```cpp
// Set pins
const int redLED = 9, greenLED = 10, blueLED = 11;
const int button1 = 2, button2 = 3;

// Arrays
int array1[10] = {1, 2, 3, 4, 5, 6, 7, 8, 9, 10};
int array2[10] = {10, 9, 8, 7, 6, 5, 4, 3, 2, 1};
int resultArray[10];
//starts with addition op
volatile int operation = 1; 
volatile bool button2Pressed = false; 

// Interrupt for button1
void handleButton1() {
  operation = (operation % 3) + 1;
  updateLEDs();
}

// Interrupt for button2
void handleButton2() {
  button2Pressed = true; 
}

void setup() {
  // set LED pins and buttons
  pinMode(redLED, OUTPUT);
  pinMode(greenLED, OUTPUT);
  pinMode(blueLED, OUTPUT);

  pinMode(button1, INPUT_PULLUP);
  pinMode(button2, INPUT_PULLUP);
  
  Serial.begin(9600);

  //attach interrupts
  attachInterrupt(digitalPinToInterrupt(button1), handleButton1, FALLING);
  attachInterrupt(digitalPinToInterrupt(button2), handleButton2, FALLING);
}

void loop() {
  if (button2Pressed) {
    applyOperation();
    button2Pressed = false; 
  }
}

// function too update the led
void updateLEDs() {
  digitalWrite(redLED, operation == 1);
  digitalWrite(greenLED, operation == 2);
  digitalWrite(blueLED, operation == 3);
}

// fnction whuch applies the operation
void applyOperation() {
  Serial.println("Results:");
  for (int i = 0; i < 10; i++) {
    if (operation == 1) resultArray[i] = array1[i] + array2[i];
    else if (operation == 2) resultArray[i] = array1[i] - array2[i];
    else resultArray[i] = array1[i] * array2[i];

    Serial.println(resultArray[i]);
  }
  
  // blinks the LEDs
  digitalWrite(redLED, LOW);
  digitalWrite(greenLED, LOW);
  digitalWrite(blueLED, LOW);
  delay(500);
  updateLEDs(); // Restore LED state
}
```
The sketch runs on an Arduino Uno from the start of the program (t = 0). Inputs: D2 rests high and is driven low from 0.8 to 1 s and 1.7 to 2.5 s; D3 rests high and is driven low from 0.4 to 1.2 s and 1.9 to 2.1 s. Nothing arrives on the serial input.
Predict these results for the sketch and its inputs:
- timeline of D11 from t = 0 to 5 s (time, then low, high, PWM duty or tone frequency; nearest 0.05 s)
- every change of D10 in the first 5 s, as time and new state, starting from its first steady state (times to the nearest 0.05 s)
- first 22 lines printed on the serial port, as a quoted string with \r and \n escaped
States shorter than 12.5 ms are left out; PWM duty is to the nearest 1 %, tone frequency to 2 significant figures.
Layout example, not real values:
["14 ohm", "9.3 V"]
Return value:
["0 s low; 1.7 s high; 1.9 s low; 2.4 s high", "0 s low; 0.8 s high; 1.7 s low", "\"Results:\\r\\n11\\r\\n11\\r\\n11\\r\\n11\\r\\n11\\r\\n11\\r\\n11\\r\\n11\\r\\n11\\r\\n11\\r\\nResults:\\r\\n10\\r\\n18\\r\\n24\\r\\n28\\r\\n30\\r\\n30\\r\\n28\\r\\n24\\r\\n18\\r\\n10\\r\\n\""]
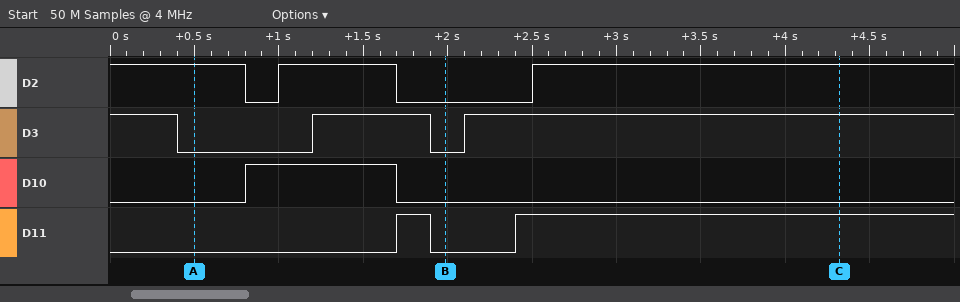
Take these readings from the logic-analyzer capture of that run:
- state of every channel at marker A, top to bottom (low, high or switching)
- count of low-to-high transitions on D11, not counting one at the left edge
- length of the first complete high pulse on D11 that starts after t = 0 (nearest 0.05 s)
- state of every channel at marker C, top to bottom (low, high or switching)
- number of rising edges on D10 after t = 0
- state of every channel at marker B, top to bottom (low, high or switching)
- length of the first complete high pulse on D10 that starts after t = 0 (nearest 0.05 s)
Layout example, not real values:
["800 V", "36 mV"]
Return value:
["D2 high, D3 low, D10 low, D11 low", "2", "0.20 s", "D2 high, D3 high, D10 low, D11 high", "1", "D2 low, D3 low, D10 low, D11 low", "0.90 s"]
